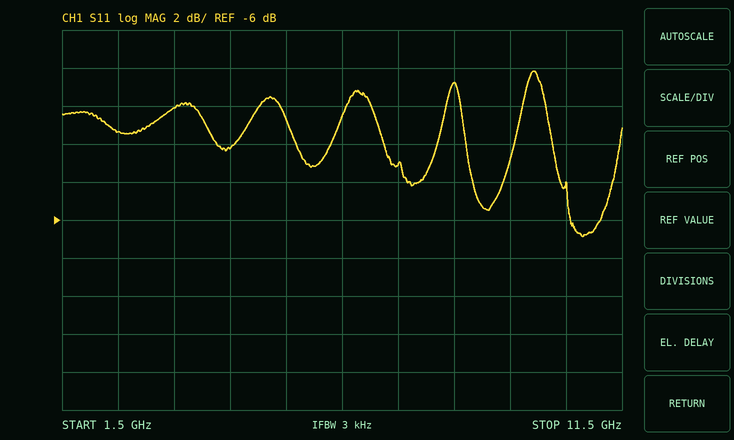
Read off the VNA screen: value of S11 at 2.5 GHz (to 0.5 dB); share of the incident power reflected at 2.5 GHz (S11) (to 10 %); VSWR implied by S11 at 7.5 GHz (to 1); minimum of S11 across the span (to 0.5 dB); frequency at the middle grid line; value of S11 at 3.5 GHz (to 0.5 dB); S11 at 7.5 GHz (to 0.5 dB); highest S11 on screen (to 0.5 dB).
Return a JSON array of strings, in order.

["-1.5 dB", "70 %", "6", "-7.0 dB", "6.5 GHz", "0.0 dB", "-3.0 dB", "2.0 dB"]
